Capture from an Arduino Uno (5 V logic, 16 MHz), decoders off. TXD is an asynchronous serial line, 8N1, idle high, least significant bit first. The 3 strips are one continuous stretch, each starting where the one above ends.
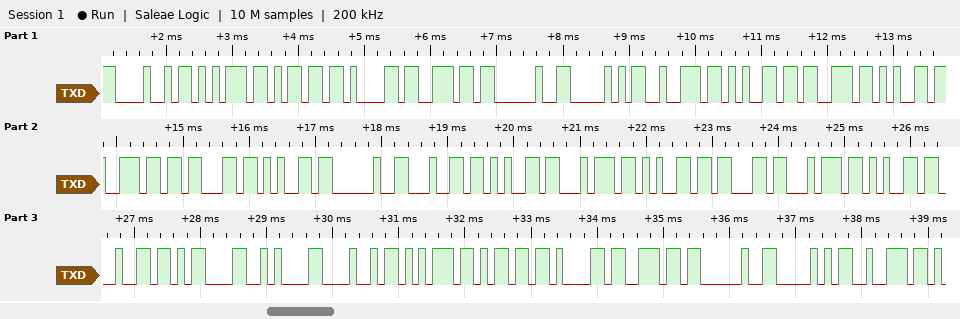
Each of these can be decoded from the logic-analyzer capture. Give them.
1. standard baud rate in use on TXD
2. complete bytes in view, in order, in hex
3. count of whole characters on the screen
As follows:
9600 baud
48 75 6D 61 6E 20 50 72 65 73 65 6E 63 65 20 64 65 74 65 63 74 65 64 0D 0A 48 75 6D 61 6E 20 50 72
33
